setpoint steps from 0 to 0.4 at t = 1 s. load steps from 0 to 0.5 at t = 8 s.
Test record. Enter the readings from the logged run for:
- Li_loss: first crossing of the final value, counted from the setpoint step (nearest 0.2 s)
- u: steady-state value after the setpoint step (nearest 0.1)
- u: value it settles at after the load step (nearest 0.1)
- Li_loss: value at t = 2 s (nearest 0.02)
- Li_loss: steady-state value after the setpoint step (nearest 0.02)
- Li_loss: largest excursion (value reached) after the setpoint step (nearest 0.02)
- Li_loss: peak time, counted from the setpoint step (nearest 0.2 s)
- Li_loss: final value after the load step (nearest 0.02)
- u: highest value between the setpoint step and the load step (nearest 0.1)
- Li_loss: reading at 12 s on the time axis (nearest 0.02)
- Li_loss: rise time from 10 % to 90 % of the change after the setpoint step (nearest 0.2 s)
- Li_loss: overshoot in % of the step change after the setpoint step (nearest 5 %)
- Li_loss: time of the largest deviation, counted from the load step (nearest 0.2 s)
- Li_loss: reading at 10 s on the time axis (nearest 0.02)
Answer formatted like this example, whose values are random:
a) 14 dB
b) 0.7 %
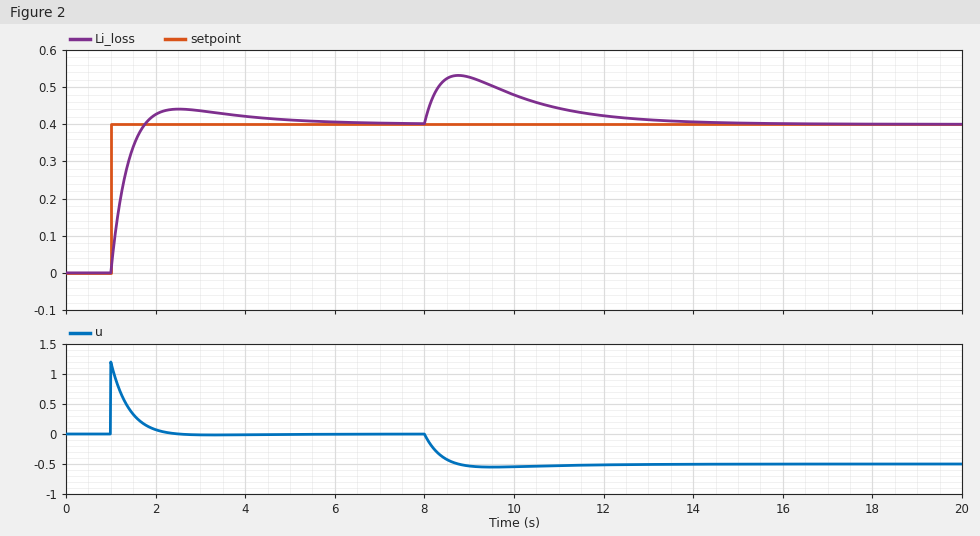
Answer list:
a) 0.8 s
b) 0.0
c) -0.5
d) 0.42
e) 0.40
f) 0.44
g) 1.6 s
h) 0.40
i) 1.2
j) 0.42
k) 0.6 s
l) 10 %
m) 0.8 s
n) 0.48
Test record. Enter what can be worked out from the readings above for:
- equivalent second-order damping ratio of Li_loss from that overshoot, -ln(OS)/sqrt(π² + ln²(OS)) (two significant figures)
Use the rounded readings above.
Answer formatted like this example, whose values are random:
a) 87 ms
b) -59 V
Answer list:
a) 0.59
